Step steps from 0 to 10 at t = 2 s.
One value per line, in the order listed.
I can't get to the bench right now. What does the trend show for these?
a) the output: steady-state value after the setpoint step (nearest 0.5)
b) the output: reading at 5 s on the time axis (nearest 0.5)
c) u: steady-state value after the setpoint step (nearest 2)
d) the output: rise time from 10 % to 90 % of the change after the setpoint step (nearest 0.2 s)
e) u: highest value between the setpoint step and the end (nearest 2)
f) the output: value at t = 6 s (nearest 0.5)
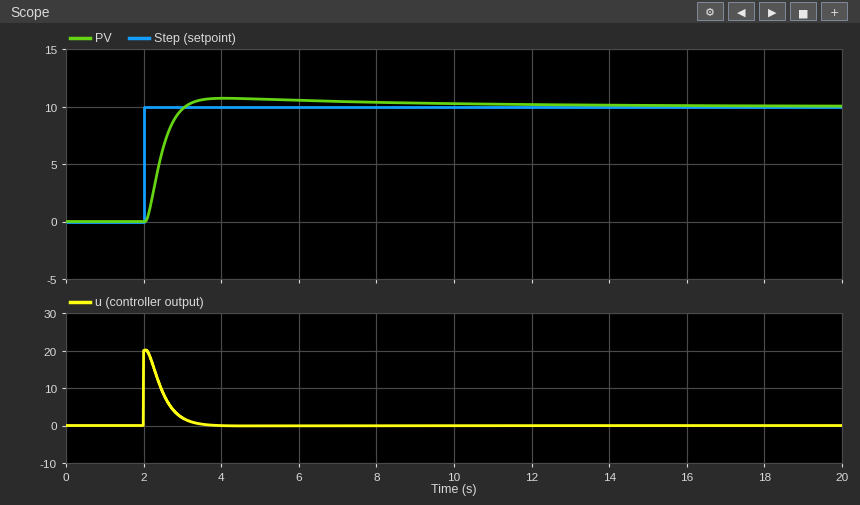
10.0
10.5
0
0.6 s
20
10.5
